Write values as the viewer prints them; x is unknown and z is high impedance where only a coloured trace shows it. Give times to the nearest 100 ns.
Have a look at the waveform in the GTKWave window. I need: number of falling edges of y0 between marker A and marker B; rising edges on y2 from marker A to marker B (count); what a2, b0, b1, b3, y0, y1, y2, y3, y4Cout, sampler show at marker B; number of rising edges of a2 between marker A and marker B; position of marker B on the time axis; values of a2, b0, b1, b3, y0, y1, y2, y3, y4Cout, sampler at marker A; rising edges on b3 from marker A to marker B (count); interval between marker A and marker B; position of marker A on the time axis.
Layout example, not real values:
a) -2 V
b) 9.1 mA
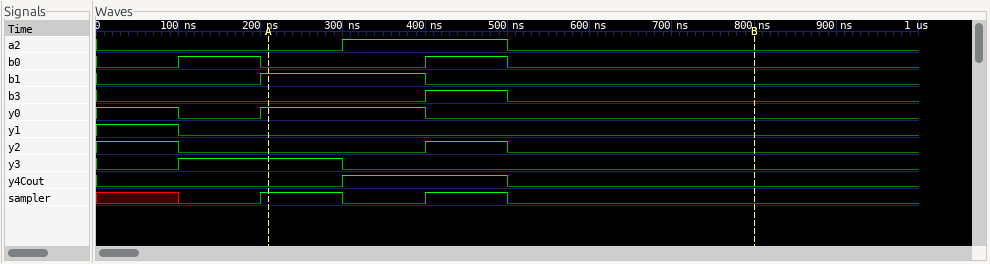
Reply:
a) 1
b) 1
c) a2=0, b0=0, b1=0, b3=0, y0=0, y1=0, y2=0, y3=0, y4Cout=0, sampler=0
d) 1
e) 800 ns
f) a2=0, b0=0, b1=1, b3=0, y0=1, y1=0, y2=0, y3=1, y4Cout=0, sampler=1
g) 1
h) 600 ns
i) 200 ns
